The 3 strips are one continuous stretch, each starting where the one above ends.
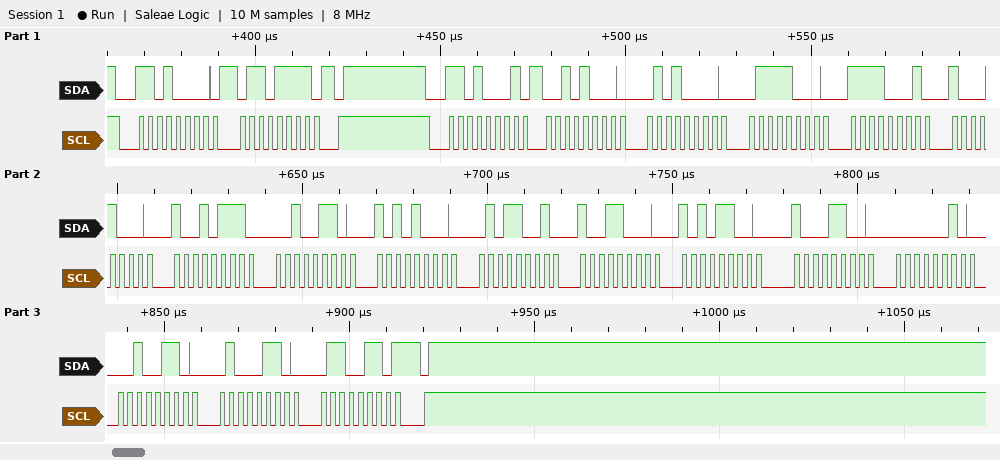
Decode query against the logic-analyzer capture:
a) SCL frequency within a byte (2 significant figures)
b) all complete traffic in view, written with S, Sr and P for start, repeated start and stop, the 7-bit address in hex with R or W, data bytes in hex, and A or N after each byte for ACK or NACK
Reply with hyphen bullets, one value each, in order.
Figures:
- 400 kHz
- S 68W A 6F A P S 68R A 28 A 50 A 78 A F1 A 88 A 97 A 26 A A8 A 59 A 98 A AC A 8C A 02 A 26 A 46 A 66 N P
